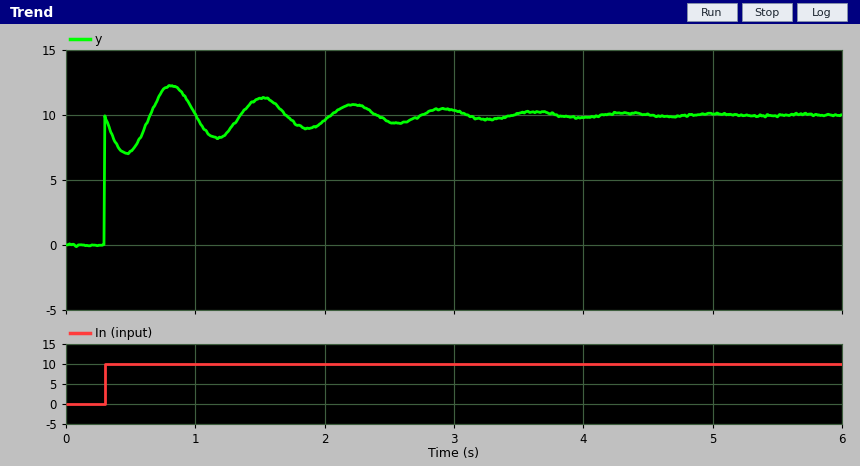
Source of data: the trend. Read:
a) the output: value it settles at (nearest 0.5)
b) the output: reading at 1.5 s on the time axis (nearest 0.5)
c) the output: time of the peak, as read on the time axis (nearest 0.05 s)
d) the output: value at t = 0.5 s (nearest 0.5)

10.0
11.5
0.80 s
7.0
